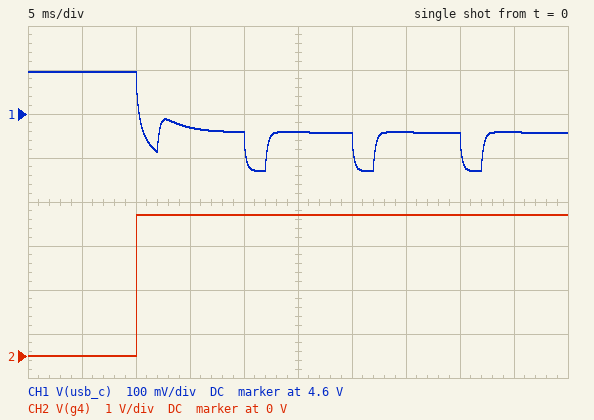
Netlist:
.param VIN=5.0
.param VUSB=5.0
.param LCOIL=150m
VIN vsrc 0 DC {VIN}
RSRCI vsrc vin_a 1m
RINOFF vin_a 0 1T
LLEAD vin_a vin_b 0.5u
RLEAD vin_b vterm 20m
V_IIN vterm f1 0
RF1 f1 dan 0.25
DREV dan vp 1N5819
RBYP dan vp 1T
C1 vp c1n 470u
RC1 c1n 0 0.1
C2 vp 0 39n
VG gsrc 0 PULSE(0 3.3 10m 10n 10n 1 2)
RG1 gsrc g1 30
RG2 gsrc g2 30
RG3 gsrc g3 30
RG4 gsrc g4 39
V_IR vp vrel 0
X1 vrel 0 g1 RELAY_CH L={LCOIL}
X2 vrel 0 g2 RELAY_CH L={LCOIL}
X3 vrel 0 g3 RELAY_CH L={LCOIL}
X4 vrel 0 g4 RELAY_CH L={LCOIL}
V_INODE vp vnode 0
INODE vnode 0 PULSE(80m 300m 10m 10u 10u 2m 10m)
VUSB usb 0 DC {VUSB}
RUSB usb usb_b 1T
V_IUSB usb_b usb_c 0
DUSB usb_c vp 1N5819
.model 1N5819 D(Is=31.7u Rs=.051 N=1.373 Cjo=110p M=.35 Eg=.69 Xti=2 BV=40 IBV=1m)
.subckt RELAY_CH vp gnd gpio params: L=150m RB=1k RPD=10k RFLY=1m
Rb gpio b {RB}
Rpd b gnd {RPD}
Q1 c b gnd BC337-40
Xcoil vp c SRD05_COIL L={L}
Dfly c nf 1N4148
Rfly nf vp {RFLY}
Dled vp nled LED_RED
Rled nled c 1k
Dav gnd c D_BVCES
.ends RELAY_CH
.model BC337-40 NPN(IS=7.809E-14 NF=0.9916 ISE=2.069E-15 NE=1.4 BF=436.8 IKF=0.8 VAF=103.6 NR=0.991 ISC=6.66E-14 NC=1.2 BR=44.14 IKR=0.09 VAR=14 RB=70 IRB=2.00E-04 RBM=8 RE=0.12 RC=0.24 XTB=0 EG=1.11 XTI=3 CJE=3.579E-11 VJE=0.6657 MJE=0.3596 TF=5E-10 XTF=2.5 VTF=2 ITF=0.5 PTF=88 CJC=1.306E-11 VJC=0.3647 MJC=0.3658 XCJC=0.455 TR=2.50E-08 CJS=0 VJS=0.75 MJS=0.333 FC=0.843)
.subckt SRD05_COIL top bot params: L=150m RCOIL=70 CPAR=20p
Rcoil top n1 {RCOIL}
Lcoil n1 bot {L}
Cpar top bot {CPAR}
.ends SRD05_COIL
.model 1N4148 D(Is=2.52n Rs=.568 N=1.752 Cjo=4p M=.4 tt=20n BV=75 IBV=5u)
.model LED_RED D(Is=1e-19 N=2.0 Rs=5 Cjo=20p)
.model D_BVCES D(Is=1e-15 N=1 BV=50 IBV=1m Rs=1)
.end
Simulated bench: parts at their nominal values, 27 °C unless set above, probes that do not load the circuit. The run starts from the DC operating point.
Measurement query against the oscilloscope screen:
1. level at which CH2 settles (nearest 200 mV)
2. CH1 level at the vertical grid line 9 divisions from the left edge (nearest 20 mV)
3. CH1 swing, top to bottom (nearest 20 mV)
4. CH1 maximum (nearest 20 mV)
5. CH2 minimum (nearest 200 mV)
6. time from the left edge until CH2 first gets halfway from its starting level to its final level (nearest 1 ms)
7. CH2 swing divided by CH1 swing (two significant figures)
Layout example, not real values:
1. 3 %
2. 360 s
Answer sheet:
1. 3.2 V
2. 4.56 V
3. 220 mV
4. 4.70 V
5. 0 V
6. 10 ms
7. 14
